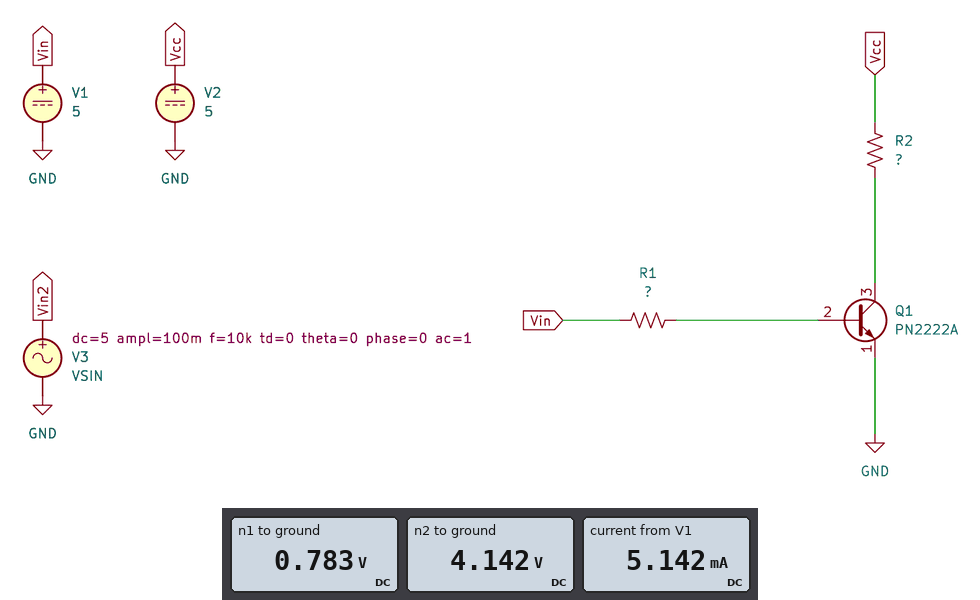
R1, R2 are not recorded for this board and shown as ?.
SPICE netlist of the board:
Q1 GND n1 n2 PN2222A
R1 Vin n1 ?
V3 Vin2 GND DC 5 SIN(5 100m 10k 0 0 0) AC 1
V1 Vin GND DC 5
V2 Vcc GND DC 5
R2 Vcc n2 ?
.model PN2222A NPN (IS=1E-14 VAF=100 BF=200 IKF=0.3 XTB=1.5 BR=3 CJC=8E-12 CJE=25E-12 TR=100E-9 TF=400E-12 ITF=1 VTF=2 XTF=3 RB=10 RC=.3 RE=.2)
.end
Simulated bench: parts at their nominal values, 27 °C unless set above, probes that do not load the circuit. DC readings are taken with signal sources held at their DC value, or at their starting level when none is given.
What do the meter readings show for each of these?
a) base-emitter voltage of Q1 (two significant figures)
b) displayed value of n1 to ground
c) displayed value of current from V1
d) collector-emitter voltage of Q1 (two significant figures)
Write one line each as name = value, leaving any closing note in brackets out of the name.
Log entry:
base-emitter voltage of Q1 = -3.4 V
displayed value of n1 to ground = 0.783 V
displayed value of current from V1 = 5.142 mA
collector-emitter voltage of Q1 = -4.1 V
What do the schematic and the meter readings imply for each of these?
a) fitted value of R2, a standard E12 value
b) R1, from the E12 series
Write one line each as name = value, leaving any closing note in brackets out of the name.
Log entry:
fitted value of R2, a standard E12 value = 56 Ω
R1, from the E12 series = 820 Ω
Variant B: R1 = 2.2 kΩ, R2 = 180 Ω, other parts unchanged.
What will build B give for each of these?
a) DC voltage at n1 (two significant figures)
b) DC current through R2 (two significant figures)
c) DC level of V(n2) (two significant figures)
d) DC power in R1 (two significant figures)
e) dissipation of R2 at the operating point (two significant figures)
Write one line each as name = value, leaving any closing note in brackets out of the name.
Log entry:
DC voltage at n1 = 720 mV
DC current through R2 = 5.8 mA
DC level of V(n2) = 4.0 V
DC power in R1 = 8.3 mW
dissipation of R2 at the operating point = 6.0 mW
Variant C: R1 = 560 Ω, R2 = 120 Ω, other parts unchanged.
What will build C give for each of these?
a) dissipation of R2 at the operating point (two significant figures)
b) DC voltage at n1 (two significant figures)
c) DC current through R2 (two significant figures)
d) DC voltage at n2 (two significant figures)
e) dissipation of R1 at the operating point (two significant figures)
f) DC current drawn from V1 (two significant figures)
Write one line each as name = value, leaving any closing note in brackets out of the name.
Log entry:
dissipation of R2 at the operating point = 59 mW
DC voltage at n1 = 820 mV
DC current through R2 = 22 mA
DC voltage at n2 = 2.3 V
dissipation of R1 at the operating point = 31 mW
DC current drawn from V1 = 7.5 mA
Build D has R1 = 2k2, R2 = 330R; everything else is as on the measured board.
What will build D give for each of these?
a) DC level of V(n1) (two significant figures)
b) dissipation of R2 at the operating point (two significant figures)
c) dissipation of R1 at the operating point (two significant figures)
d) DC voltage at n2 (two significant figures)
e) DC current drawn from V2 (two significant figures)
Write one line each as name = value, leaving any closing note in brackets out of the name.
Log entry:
DC level of V(n1) = 720 mV
dissipation of R2 at the operating point = 11 mW
dissipation of R1 at the operating point = 8.3 mW
DC voltage at n2 = 3.1 V
DC current drawn from V2 = 5.8 mA
